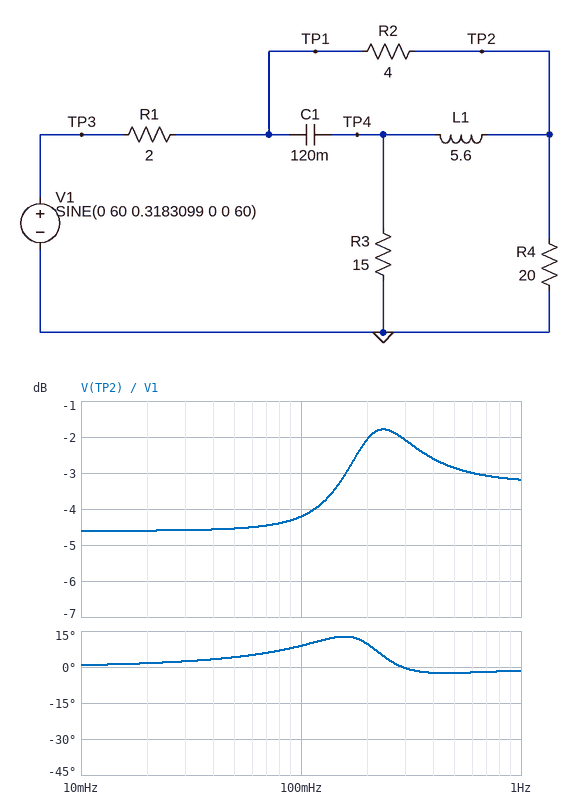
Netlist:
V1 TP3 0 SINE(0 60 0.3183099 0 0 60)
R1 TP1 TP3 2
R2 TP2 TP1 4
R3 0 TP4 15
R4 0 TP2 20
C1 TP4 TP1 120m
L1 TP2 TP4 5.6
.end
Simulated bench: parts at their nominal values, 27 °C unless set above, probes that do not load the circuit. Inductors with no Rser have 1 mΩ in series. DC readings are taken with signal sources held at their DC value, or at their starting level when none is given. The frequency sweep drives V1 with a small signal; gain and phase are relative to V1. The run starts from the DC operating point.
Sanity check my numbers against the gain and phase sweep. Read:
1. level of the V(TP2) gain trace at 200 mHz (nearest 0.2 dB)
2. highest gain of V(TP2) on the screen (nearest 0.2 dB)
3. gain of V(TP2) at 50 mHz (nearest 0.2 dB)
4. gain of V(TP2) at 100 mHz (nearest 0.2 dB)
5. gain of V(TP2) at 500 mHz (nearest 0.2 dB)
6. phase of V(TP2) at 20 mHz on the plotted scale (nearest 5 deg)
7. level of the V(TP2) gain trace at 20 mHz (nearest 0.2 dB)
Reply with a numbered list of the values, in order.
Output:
1. -2.0 dB
2. -1.8 dB
3. -4.6 dB
4. -4.2 dB
5. -2.8 dB
6. 0 deg
7. -4.6 dB
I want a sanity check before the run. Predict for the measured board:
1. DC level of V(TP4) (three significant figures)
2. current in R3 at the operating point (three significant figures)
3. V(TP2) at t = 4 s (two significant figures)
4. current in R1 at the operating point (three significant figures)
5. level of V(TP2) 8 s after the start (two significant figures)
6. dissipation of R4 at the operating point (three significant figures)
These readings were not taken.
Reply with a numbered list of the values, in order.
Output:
1. 30.6 V
2. 2.04 A
3. 19 V
4. 3.57 A
5. -45 V
6. 46.7 W
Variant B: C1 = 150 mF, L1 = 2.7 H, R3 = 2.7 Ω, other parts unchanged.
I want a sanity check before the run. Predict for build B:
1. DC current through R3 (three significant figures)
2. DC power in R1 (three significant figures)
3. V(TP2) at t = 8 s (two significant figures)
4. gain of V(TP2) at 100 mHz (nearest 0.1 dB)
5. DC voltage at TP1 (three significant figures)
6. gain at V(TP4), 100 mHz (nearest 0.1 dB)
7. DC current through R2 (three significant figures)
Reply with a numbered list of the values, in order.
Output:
1. 5.46 A
2. 76.9 W
3. -41 V
4. -8.6 dB
5. 39.6 V
6. -11.9 dB
7. 6.20 A
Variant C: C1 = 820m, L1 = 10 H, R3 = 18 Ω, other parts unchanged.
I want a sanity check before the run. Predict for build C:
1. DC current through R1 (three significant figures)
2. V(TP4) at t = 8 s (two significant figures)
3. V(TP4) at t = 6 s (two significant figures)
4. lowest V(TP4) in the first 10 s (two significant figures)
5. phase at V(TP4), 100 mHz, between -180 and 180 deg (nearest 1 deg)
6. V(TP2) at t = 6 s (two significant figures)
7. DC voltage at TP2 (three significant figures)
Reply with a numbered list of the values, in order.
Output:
1. 3.36 A
2. -47 V
3. 26 V
4. -57 V
5. 9 deg
6. 15 V
7. 31.8 V
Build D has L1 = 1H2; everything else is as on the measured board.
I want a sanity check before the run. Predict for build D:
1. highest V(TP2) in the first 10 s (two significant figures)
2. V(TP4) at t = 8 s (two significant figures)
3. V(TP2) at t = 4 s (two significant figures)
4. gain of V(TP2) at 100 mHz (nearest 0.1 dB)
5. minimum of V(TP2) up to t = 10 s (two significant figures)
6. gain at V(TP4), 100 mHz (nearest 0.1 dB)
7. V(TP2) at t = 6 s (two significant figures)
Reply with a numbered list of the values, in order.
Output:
1. 44 V
2. -37 V
3. 8.2 V
4. -4.4 dB
5. -44 V
6. -4.7 dB
7. 27 V
